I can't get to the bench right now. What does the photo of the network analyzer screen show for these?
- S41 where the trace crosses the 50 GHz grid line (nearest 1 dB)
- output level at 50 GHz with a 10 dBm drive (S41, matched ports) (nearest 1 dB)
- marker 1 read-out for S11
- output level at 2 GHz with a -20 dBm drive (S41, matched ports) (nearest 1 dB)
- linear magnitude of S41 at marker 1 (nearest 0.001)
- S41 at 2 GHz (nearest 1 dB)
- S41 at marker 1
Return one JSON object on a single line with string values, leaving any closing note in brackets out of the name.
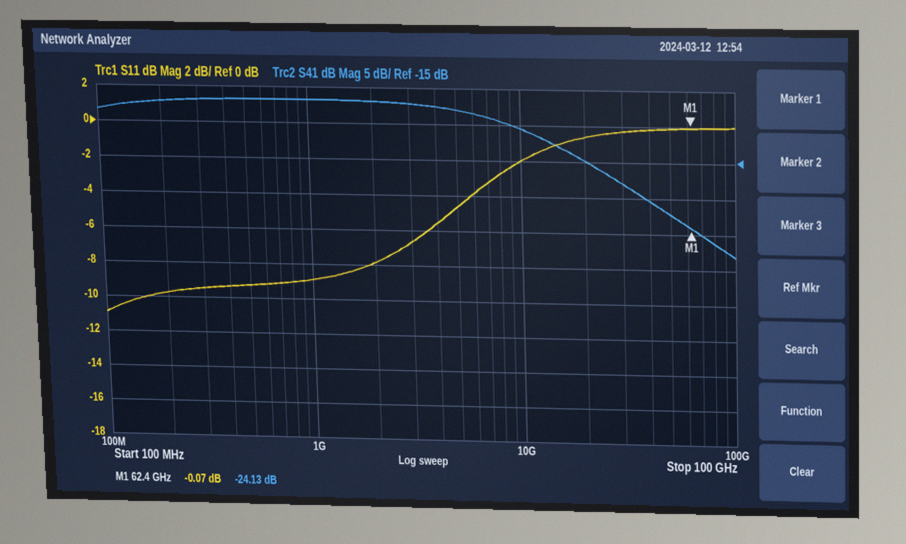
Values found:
{"S41 where the trace crosses the 50 GHz grid line": "-22 dB", "output level at 50 GHz with a 10 dBm drive (S41, matched ports)": "-12 dBm", "marker 1 read-out for S11": "-0.07 dB", "output level at 2 GHz with a -20 dBm drive (S41, matched ports)": "-27 dBm", "linear magnitude of S41 at marker 1": "0.062", "S41 at 2 GHz": "-7 dB", "S41 at marker 1": "-24.13 dB"}
